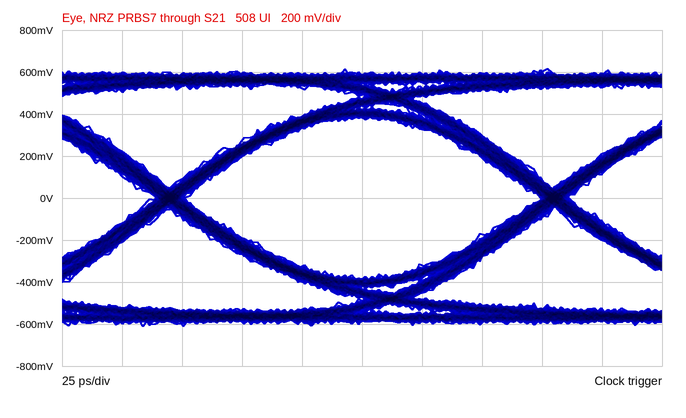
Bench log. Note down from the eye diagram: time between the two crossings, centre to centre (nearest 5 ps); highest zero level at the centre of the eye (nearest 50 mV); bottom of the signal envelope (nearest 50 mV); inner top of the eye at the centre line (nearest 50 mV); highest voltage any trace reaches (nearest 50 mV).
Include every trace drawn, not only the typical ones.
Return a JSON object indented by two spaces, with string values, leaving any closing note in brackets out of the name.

{
  "time between the two crossings, centre to centre": "160 ps",
  "highest zero level at the centre of the eye": "-400 mV",
  "bottom of the signal envelope": "-600 mV",
  "inner top of the eye at the centre line": "400 mV",
  "highest voltage any trace reaches": "600 mV"
}
